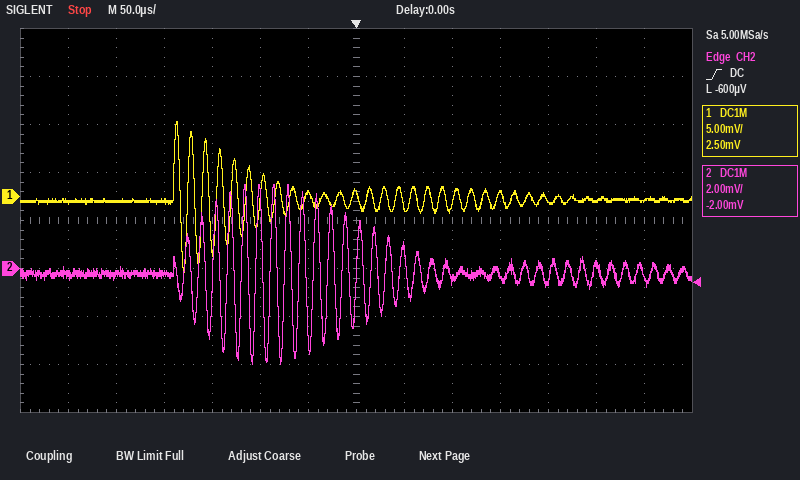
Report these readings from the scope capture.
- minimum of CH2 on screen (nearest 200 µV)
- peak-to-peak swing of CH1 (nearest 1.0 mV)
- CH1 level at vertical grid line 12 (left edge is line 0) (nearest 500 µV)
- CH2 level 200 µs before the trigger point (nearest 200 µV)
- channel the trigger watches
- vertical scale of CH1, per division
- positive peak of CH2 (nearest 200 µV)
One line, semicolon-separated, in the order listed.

-4.0 mV; 16.0 mV; -500 µV; -200 µV; CH2; 5 mV; 3.6 mV
